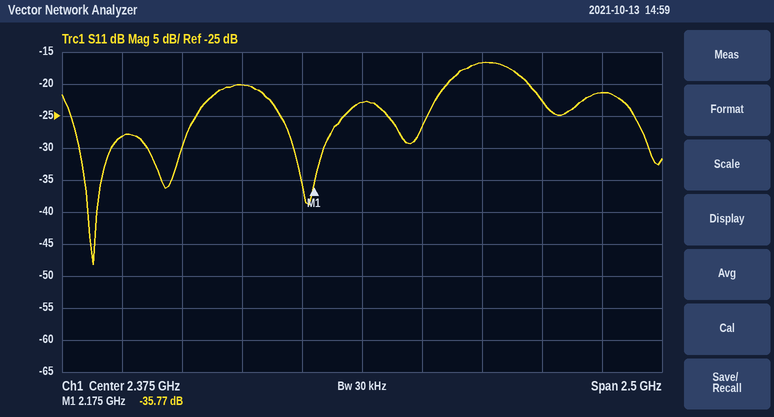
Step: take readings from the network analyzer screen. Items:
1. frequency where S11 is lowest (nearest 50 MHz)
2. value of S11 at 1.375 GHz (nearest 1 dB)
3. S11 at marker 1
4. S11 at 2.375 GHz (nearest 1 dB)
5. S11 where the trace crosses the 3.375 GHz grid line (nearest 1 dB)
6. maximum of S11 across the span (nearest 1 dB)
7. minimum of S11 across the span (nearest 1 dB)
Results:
1.25 GHz
-28 dB
-35.77 dB
-23 dB
-21 dB
-17 dB
-48 dB
